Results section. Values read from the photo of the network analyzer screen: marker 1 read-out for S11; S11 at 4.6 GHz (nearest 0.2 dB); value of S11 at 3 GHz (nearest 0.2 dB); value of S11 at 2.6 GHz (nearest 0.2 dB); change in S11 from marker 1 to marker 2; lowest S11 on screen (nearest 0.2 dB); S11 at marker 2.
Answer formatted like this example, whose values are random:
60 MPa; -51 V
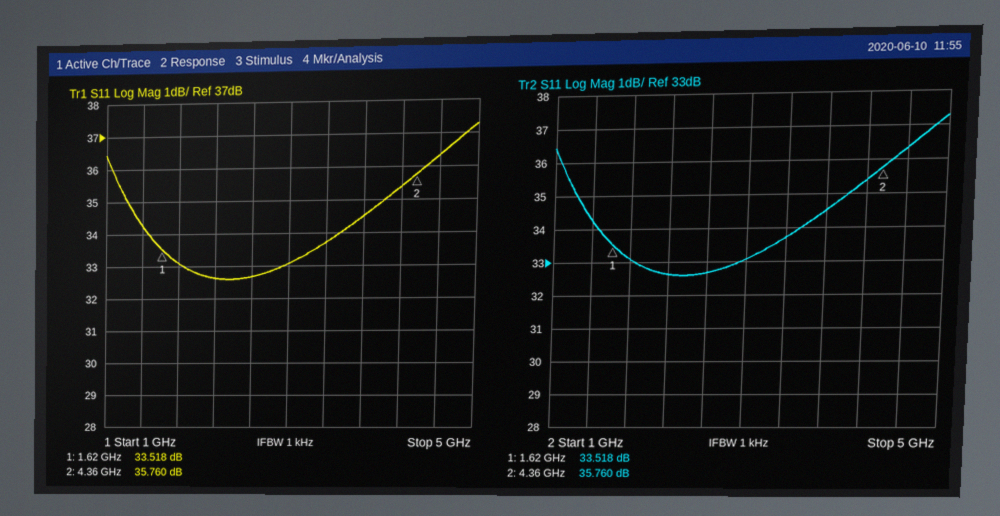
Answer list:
33.518 dB; 36.4 dB; 33.0 dB; 32.6 dB; 2.242 dB; 32.6 dB; 35.760 dB
